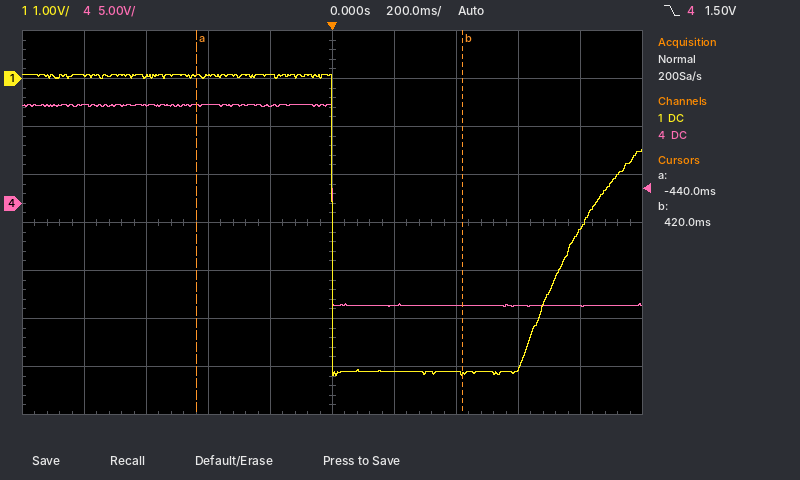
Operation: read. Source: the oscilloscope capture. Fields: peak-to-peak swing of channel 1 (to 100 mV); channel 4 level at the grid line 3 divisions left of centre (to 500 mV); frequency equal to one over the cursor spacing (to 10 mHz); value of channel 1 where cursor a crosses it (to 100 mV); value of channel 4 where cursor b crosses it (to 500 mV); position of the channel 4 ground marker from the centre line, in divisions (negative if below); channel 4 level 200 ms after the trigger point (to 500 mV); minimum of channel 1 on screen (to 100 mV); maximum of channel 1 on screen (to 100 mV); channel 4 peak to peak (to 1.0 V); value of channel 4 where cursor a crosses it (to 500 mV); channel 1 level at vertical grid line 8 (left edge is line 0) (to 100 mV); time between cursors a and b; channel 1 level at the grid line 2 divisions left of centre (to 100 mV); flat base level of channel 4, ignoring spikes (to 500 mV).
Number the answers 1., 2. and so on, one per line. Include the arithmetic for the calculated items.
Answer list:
1. 100 mV − (-6.2 V) = 6.3 V
2. 10.0 V
3. 1 / 860 ms ≈ 1.16 Hz
4. 100 mV
5. -10.5 V
6. +0.4 div
7. -10.5 V
8. -6.2 V
9. 100 mV
10. 21.0 V
11. 10.0 V
12. -6.0 V
13. 420 ms − (-440 ms) = 860 ms
14. 100 mV
15. -10.5 V
